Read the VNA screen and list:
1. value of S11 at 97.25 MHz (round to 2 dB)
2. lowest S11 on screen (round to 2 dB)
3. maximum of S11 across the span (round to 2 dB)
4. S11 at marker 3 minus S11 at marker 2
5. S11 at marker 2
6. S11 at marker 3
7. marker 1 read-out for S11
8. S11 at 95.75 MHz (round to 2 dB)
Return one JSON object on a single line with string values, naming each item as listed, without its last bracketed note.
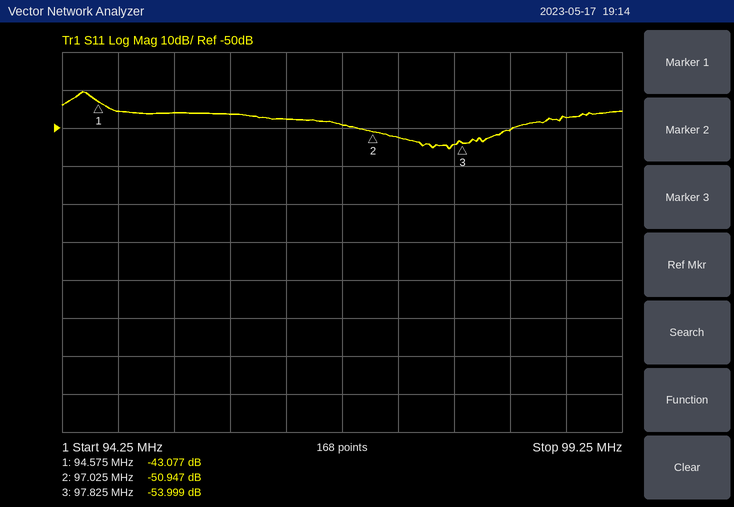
{"value of S11 at 97.25 MHz": "-52 dB", "lowest S11 on screen": "-56 dB", "maximum of S11 across the span": "-40 dB", "S11 at marker 3 minus S11 at marker 2": "-3.052 dB", "S11 at marker 2": "-50.947 dB", "S11 at marker 3": "-53.999 dB", "marker 1 read-out for S11": "-43.077 dB", "S11 at 95.75 MHz": "-46 dB"}
